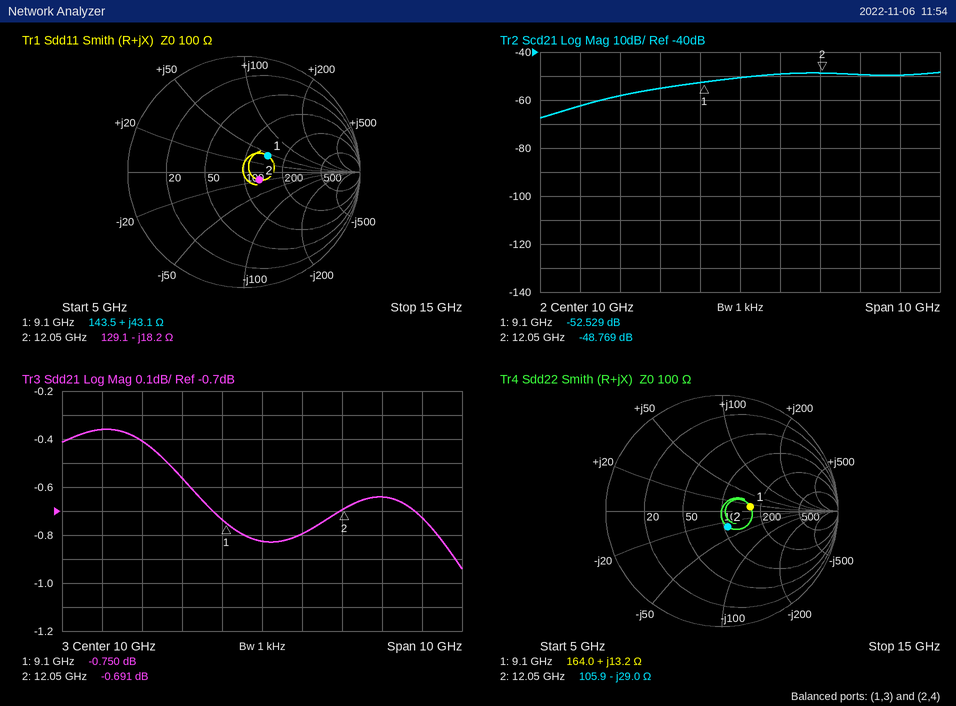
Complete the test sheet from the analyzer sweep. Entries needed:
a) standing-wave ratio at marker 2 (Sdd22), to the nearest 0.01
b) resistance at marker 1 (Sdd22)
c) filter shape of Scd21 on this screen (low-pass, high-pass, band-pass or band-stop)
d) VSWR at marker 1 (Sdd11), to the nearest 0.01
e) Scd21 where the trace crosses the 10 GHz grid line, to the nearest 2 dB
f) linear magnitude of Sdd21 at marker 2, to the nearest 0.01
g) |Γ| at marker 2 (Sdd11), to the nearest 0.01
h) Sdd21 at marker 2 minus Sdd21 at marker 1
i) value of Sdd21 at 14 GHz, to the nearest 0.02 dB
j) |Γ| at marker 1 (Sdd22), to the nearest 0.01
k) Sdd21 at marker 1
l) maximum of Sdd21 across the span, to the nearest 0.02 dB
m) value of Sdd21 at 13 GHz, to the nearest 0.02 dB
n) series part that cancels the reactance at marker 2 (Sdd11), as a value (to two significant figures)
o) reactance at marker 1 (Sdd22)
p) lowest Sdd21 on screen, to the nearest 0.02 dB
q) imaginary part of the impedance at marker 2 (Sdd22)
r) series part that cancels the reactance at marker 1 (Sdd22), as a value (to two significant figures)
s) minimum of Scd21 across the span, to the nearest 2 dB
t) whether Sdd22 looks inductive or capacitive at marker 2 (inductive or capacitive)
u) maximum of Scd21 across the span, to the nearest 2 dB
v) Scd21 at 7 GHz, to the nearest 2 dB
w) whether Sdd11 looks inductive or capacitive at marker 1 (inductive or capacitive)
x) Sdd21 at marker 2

1.33
164.0 Ω
high-pass
1.66
-50 dB
0.92
0.15
0.059 dB
-0.72 dB
0.25
-0.750 dB
-0.36 dB
-0.64 dB
240 pH
+13.2 Ω
-0.94 dB
-29.0 Ω
1.3 pF
-68 dB
capacitive
-48 dB
-58 dB
inductive
-0.691 dB
